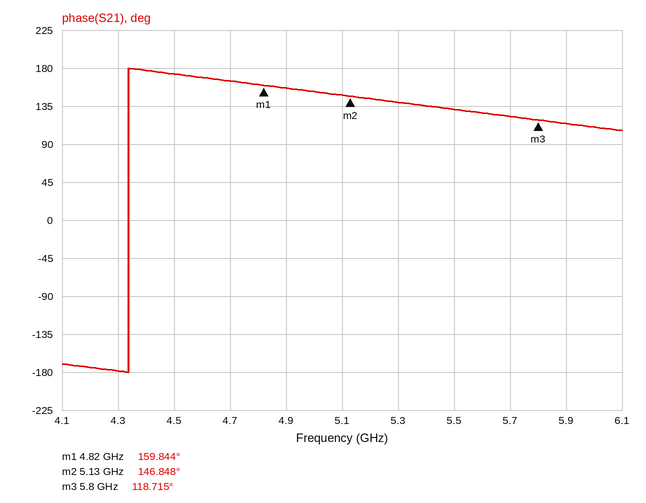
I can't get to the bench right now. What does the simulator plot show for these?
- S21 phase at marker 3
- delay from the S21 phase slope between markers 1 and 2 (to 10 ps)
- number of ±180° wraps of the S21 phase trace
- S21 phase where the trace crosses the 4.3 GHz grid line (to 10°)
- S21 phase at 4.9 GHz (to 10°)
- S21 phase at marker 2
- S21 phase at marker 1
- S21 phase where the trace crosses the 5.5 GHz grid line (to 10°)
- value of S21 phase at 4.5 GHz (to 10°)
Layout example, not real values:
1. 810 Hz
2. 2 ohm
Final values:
1. 118.715°
2. 120 ps
3. 1
4. -180°
5. 160°
6. 146.848°
7. 159.844°
8. 130°
9. 170°
